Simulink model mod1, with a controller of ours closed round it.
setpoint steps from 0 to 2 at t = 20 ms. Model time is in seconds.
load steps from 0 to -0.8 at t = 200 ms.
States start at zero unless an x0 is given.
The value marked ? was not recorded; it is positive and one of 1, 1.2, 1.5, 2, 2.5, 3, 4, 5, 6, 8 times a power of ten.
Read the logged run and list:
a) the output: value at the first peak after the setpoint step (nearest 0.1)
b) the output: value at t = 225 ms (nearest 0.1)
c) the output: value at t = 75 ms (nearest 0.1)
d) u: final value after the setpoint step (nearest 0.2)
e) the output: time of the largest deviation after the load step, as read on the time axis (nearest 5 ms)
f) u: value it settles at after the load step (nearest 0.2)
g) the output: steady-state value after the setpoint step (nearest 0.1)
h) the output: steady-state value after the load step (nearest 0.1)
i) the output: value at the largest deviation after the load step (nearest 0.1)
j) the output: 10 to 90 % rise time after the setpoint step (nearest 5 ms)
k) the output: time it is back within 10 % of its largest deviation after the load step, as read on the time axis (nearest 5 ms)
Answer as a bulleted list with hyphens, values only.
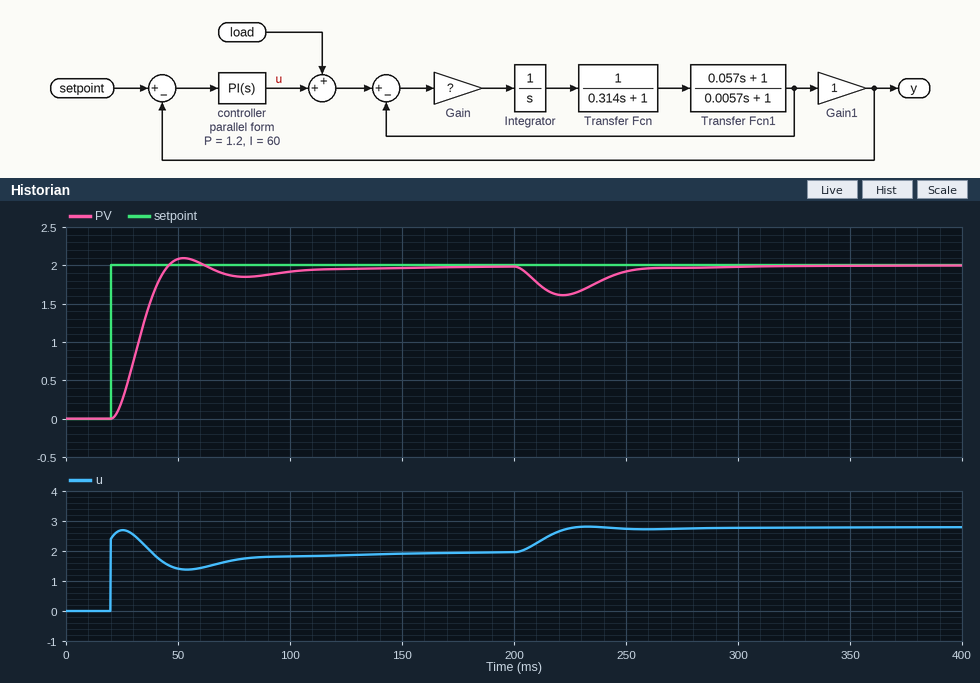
- 2.1
- 1.6
- 1.9
- 2.0
- 220 ms
- 2.8
- 2.0
- 2.0
- 1.6
- 15 ms
- 260 ms
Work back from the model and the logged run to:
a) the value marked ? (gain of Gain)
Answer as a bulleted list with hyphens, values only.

- 300
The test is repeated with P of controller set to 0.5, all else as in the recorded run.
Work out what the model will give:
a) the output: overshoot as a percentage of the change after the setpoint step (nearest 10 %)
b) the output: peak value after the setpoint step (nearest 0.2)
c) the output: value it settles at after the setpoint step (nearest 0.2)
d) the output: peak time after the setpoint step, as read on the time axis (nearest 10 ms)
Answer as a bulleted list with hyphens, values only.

- 20 %
- 2.4
- 2.0
- 70 ms
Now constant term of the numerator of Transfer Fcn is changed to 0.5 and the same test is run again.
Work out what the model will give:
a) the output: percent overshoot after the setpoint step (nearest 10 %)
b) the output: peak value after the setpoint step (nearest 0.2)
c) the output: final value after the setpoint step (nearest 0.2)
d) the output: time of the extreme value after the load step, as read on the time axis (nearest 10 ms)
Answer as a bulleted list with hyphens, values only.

- 20 %
- 2.4
- 2.0
- 230 ms
